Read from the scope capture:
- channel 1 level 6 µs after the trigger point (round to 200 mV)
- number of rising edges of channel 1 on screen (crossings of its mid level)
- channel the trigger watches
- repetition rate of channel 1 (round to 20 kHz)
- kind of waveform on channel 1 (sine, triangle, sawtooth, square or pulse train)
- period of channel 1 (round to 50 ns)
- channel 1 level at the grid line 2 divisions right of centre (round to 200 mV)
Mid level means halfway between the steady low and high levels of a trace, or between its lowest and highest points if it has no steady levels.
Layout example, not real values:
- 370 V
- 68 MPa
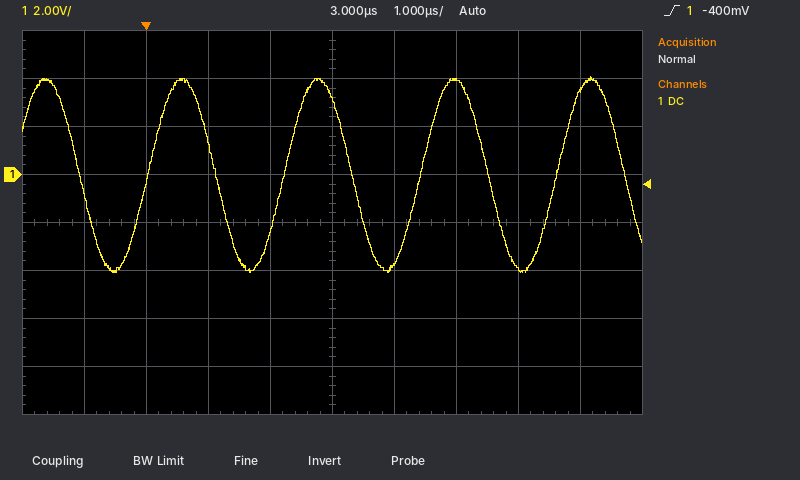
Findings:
- -4.0 V
- 4
- channel 1
- 460 kHz
- sine
- 2.20 µs
- 4.0 V
